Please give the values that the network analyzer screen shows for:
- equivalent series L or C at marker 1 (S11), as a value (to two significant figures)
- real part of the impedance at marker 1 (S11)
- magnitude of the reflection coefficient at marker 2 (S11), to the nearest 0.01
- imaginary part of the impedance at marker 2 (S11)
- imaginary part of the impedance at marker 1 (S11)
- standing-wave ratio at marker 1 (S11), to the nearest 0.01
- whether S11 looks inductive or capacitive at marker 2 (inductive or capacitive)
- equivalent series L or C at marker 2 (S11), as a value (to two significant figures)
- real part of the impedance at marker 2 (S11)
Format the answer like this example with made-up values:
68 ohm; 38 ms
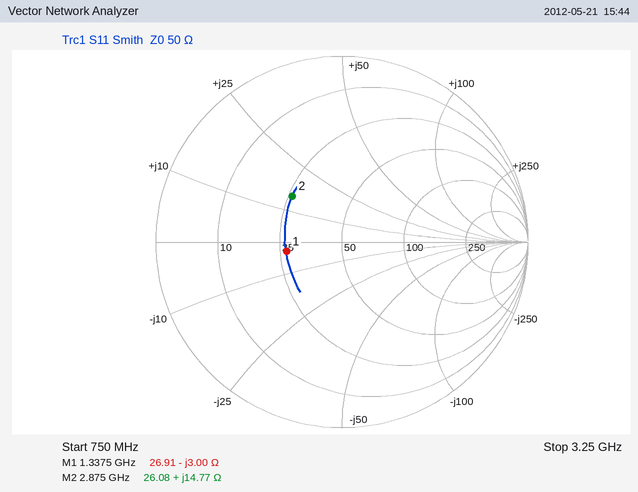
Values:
40 pF; 26.91 Ω; 0.36; +14.77 Ω; -3.00 Ω; 1.87; inductive; 820 pH; 26.08 Ω
